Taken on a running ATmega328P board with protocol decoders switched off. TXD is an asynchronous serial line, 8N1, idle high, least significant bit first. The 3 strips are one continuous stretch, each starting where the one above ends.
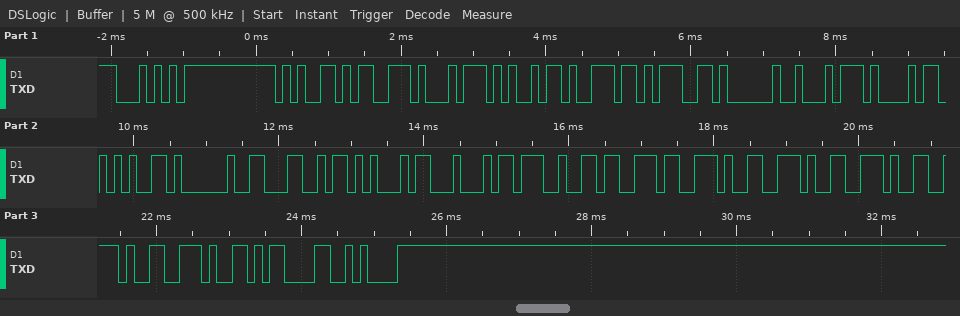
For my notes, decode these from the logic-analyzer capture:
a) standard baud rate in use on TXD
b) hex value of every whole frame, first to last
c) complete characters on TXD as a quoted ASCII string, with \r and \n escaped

9600 baud
54 65 73 74 69 6E 67 20 74 68 65 20 4C 45 44 27 73 2E 2E 2E 2E 2E 0D 0A
"Testing the LED's.....\r\n"
